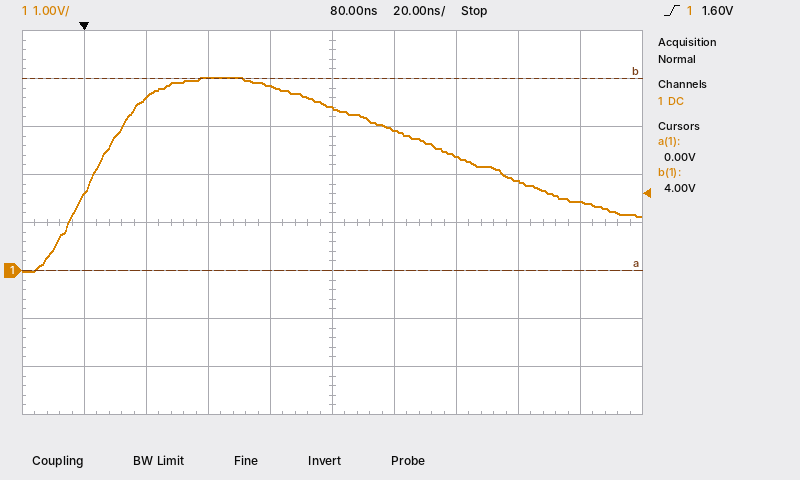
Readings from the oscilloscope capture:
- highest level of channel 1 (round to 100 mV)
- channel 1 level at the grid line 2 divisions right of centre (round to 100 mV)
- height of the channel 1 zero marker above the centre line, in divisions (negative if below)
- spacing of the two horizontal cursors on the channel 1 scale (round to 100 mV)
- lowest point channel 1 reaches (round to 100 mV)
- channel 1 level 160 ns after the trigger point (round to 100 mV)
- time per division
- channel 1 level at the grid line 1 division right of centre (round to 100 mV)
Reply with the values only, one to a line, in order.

4.0 V
2.4 V
-1.0 div
4.0 V
0.0 V
1.4 V
20 ns
2.9 V
